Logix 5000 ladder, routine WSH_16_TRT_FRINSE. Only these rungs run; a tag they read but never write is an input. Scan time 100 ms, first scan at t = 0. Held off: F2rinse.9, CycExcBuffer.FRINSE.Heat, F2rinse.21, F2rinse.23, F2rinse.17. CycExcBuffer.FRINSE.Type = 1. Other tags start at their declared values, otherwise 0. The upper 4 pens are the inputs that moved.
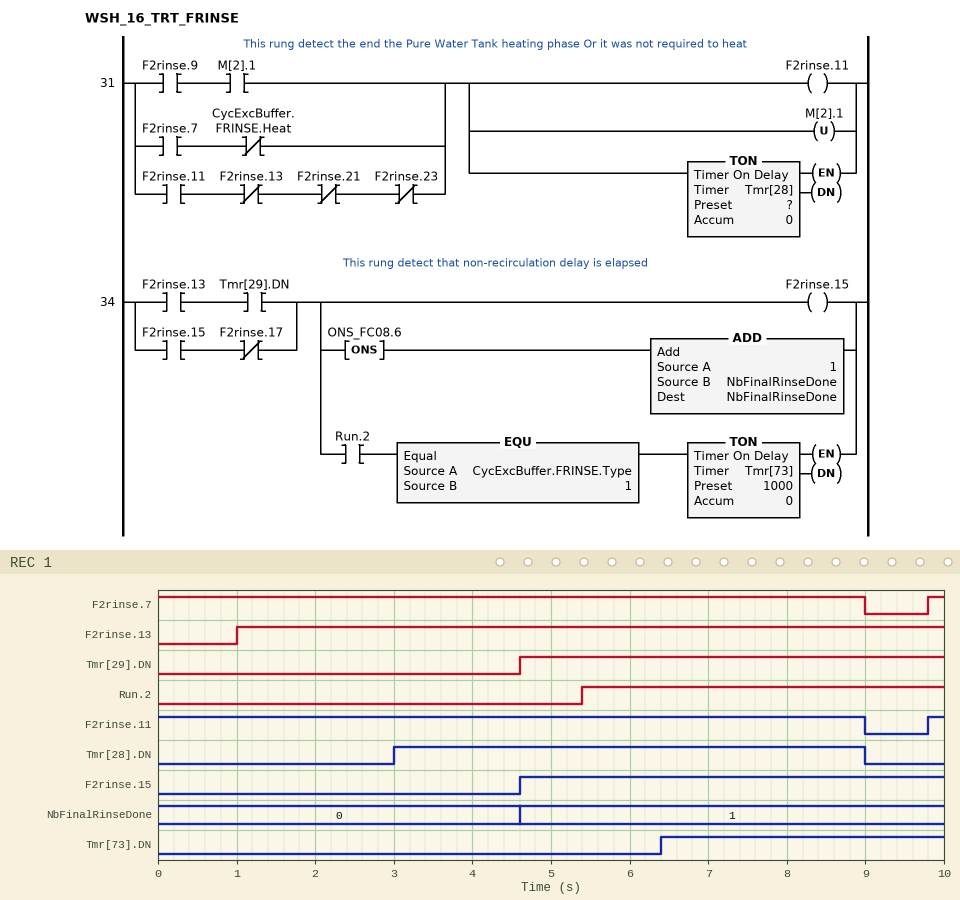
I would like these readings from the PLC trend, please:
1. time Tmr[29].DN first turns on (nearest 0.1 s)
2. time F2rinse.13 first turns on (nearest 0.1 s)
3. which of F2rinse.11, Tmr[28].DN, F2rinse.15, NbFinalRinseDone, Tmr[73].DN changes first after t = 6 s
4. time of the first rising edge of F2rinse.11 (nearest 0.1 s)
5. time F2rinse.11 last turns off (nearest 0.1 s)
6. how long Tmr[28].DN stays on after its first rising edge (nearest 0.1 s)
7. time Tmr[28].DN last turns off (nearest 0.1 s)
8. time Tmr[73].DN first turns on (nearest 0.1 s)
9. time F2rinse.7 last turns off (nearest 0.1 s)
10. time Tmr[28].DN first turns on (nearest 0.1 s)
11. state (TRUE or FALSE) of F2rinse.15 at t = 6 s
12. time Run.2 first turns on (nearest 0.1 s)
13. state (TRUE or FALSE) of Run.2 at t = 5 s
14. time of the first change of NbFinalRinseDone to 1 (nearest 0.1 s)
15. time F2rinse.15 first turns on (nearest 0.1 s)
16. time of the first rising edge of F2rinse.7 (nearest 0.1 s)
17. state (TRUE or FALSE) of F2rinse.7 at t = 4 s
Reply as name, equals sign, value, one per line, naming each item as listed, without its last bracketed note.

time Tmr[29].DN first turns on = 4.6 s
time F2rinse.13 first turns on = 1.0 s
which of F2rinse.11, Tmr[28].DN, F2rinse.15, NbFinalRinseDone, Tmr[73].DN changes first after t = 6 s = Tmr[73].DN
time of the first rising edge of F2rinse.11 = 9.8 s
time F2rinse.11 last turns off = 9.0 s
how long Tmr[28].DN stays on after its first rising edge = 6.0 s
time Tmr[28].DN last turns off = 9.0 s
time Tmr[73].DN first turns on = 6.4 s
time F2rinse.7 last turns off = 9.0 s
time Tmr[28].DN first turns on = 3.0 s
state (TRUE or FALSE) of F2rinse.15 at t = 6 s = TRUE
time Run.2 first turns on = 5.4 s
state (TRUE or FALSE) of Run.2 at t = 5 s = FALSE
time of the first change of NbFinalRinseDone to 1 = 4.6 s
time F2rinse.15 first turns on = 4.6 s
time of the first rising edge of F2rinse.7 = 9.8 s
state (TRUE or FALSE) of F2rinse.7 at t = 4 s = TRUE
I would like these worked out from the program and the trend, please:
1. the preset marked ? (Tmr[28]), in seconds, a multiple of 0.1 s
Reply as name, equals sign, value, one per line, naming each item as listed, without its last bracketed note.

the preset marked ? (Tmr[28]), in seconds, a multiple of 0.1 s = 3.0 s
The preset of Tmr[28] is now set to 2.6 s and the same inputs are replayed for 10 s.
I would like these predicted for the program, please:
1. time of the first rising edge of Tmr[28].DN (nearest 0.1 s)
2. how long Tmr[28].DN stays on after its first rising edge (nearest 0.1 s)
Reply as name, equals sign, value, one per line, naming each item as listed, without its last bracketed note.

time of the first rising edge of Tmr[28].DN = 2.6 s
how long Tmr[28].DN stays on after its first rising edge = 6.4 s
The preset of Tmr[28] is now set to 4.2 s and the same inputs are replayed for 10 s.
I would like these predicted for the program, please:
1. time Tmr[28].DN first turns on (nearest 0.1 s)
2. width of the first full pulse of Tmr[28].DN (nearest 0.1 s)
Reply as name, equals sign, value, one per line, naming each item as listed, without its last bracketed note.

time Tmr[28].DN first turns on = 4.2 s
width of the first full pulse of Tmr[28].DN = 4.8 s
